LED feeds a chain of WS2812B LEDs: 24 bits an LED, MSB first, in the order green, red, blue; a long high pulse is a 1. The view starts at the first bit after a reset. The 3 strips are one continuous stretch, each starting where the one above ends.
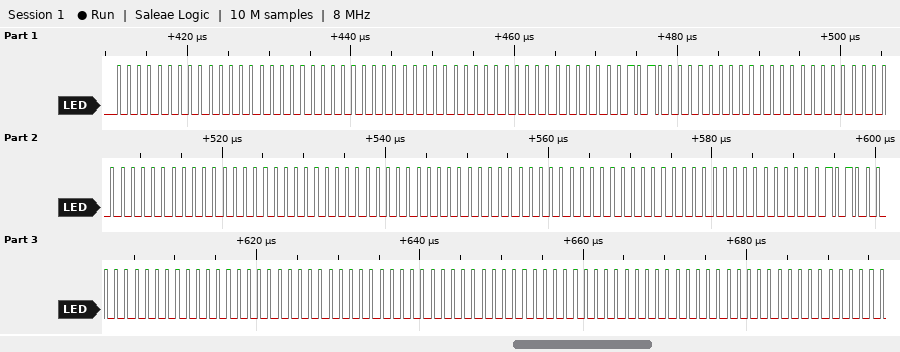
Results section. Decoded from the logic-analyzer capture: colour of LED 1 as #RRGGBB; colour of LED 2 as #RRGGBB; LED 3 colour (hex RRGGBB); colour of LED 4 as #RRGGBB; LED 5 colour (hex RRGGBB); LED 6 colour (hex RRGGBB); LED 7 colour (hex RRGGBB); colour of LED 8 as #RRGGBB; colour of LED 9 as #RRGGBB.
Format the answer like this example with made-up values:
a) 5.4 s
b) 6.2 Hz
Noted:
a) #000000
b) #000000
c) #002800
d) #000000
e) #000000
f) #000000
g) #002800
h) #000000
i) #000000
